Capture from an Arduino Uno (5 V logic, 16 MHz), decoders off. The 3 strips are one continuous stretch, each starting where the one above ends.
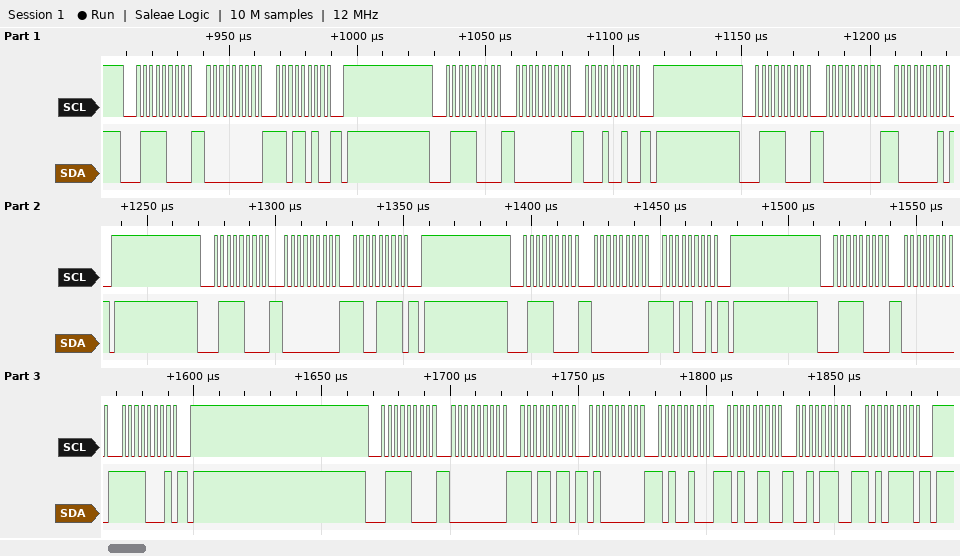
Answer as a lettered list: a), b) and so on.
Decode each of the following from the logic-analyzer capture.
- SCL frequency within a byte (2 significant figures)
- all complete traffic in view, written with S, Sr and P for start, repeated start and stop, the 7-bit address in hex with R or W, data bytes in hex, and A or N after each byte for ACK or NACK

a) 400 kHz
b) S 3CW A 00 A DA A P S 3CW A 00 A 12 A P S 3CW A 00 A 81 A P S 3CW A 00 A CF A P S 3CW A 00 A D9 A P S 3CW A 00 A F1 A P S 3CW A 00 A DB A 40 A A4 A A6 A 2E A AF A P
